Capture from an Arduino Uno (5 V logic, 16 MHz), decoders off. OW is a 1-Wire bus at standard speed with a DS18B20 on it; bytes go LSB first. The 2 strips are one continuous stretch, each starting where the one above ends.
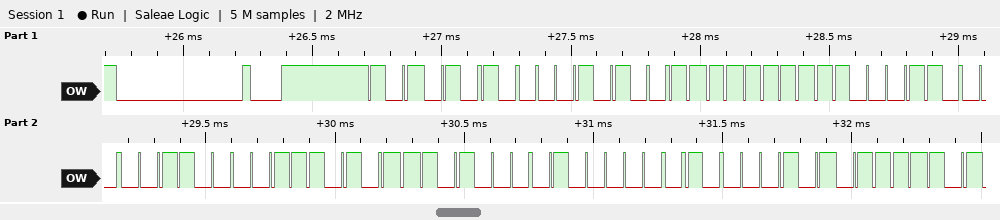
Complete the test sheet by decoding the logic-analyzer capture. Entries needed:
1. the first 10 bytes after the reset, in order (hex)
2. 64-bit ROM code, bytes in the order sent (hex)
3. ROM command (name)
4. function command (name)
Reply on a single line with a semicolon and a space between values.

55 28 FF 63 30 5C 17 02 A1 BE; 28 FF 63 30 5C 17 02 A1; Match ROM; Read Scratchpad
